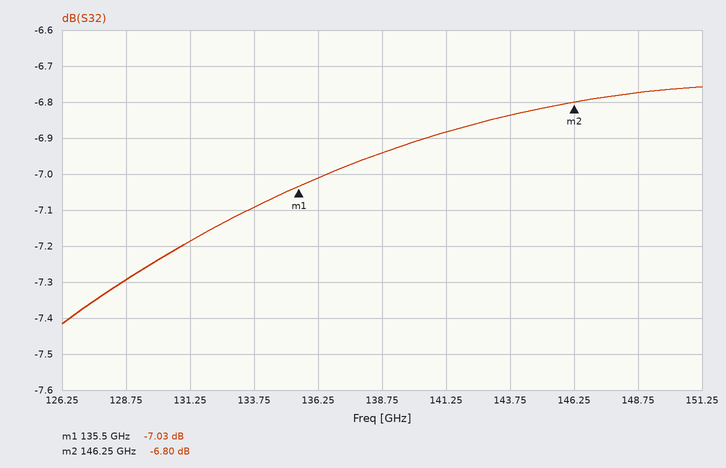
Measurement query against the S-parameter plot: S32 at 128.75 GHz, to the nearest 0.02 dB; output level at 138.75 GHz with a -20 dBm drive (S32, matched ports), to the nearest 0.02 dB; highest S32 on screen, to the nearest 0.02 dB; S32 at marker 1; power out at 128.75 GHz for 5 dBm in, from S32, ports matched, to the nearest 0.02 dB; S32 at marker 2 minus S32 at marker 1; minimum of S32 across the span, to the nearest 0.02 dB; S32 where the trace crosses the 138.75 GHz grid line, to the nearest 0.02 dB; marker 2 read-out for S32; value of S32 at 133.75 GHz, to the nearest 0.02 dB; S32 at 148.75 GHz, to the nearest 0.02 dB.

-7.30 dB
-26.94 dBm
-6.76 dB
-7.03 dB
-2.30 dBm
0.23 dB
-7.42 dB
-6.94 dB
-6.80 dB
-7.10 dB
-6.78 dB
